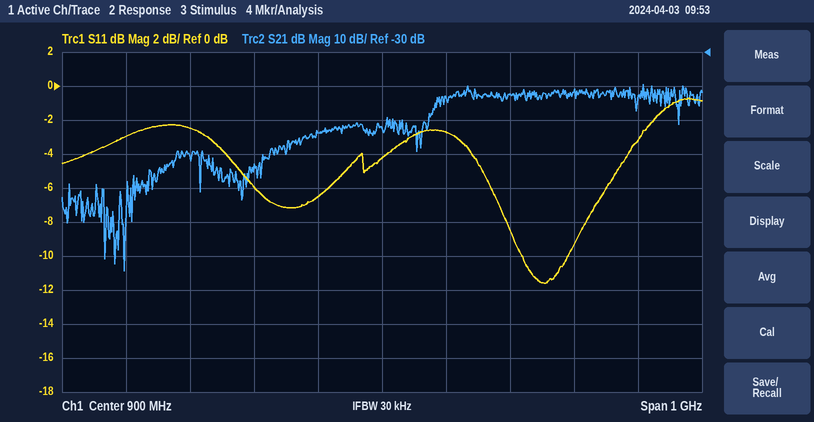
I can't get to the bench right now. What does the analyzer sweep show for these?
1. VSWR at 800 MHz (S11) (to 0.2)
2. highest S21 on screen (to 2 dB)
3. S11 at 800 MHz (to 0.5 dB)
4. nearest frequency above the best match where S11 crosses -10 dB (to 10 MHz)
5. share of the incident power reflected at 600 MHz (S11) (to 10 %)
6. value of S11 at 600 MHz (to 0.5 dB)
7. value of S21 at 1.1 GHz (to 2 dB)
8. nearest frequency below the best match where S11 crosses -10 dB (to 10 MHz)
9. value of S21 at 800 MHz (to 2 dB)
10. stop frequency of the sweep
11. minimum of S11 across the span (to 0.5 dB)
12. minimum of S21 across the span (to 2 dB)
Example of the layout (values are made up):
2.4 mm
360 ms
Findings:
2.8
-40 dB
-6.5 dB
1.19 GHz
60 %
-2.5 dB
-42 dB
1.12 GHz
-54 dB
1.4 GHz
-11.5 dB
-94 dB
